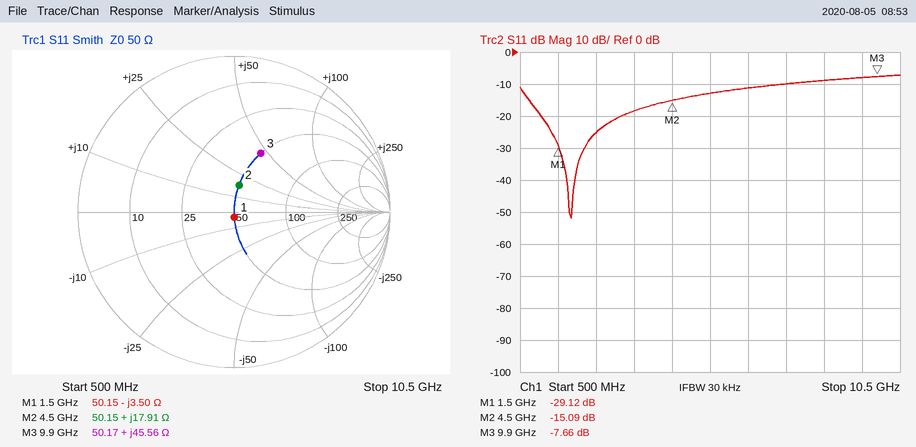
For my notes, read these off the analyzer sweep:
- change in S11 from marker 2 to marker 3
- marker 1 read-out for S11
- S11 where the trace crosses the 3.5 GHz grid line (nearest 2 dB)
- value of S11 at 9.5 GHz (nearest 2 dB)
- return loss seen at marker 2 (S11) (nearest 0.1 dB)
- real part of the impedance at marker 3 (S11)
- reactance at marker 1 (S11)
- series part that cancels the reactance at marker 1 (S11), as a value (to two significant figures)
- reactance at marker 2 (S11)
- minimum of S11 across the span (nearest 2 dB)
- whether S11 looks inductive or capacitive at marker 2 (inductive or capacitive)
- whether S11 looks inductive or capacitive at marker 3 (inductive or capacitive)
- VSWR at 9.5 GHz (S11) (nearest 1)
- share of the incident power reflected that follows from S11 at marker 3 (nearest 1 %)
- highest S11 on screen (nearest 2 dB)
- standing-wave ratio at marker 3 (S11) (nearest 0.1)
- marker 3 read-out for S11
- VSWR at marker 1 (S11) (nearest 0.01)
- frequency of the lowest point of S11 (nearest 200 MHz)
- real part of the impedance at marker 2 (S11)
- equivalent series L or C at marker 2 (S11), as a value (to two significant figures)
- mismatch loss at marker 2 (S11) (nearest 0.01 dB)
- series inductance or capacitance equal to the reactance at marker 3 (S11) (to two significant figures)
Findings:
7.43 dB
-29.12 dB
-18 dB
-8 dB
15.1 dB
50.17 Ω
-3.50 Ω
370 pH
+17.91 Ω
-52 dB
inductive
inductive
2
17 %
-8 dB
2.4
-7.66 dB
1.07
1.8 GHz
50.15 Ω
630 pH
0.14 dB
730 pH
